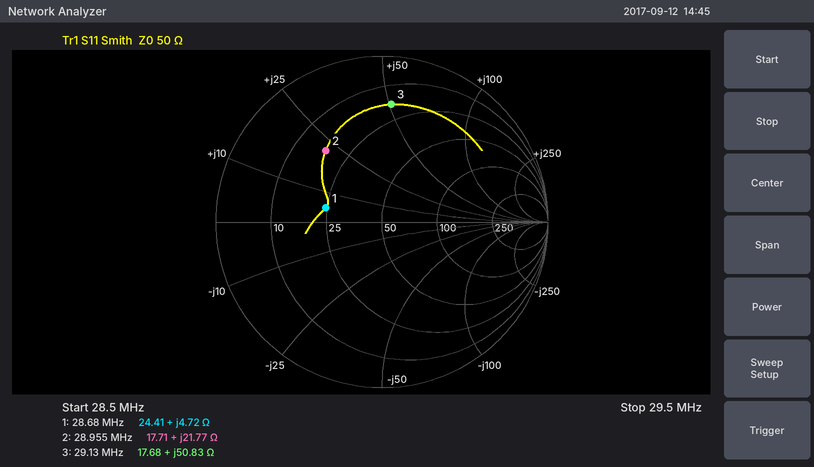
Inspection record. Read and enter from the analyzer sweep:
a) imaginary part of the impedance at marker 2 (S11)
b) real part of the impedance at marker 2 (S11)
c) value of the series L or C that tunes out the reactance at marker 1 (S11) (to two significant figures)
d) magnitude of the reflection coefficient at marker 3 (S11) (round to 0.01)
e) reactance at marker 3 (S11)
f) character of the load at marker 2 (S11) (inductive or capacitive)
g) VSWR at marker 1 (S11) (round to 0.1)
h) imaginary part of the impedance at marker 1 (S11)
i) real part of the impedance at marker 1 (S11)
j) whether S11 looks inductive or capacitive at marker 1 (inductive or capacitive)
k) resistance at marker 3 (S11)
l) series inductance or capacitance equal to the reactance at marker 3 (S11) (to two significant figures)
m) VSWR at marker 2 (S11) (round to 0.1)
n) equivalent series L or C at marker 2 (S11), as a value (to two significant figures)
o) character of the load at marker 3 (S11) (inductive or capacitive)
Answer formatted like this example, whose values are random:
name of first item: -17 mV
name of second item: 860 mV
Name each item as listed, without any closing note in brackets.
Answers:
imaginary part of the impedance at marker 2: +21.77 Ω
real part of the impedance at marker 2: 17.71 Ω
value of the series L or C that tunes out the reactance at marker 1 (S11): 1.2 nF
magnitude of the reflection coefficient at marker 3 (S11): 0.71
reactance at marker 3: +50.83 Ω
character of the load at marker 2 (S11): inductive
VSWR at marker 1 (S11): 2.1
imaginary part of the impedance at marker 1: +4.72 Ω
real part of the impedance at marker 1: 24.41 Ω
whether S11 looks inductive or capacitive at marker 1: inductive
resistance at marker 3: 17.68 Ω
series inductance or capacitance equal to the reactance at marker 3 (S11): 280 nH
VSWR at marker 2 (S11): 3.4
equivalent series L or C at marker 2 (S11), as a value: 120 nH
character of the load at marker 3 (S11): inductive
